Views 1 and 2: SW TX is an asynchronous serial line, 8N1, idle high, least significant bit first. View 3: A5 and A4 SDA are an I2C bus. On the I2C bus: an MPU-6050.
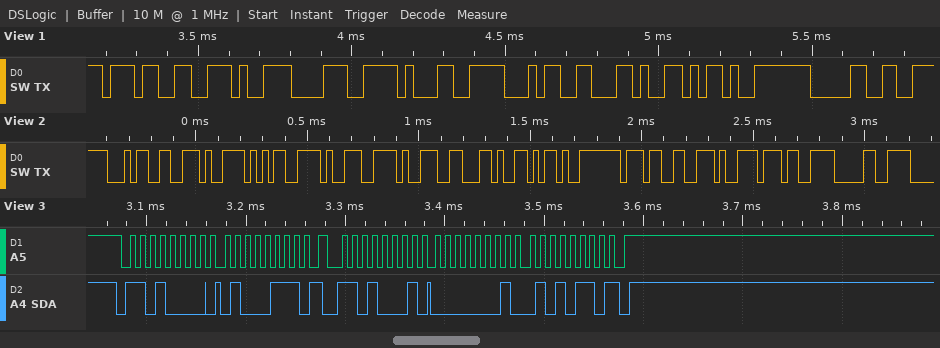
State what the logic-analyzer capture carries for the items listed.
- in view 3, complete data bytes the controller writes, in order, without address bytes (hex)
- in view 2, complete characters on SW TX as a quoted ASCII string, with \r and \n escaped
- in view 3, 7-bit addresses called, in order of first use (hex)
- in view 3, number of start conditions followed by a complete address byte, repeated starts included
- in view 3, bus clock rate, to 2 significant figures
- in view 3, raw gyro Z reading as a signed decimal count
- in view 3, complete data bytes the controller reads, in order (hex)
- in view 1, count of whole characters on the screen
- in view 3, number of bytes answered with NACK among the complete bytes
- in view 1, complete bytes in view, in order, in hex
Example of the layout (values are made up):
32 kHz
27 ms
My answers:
47
"4.599,-7.70"
0x68
2
100 kHz
342
01 56
8
1
37 2E 38 31 34 2C 2D 30
